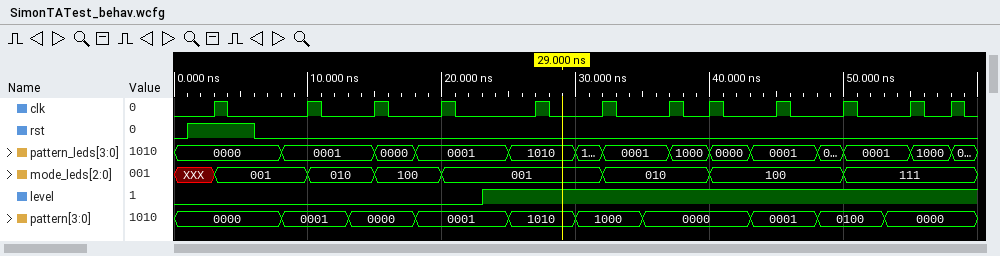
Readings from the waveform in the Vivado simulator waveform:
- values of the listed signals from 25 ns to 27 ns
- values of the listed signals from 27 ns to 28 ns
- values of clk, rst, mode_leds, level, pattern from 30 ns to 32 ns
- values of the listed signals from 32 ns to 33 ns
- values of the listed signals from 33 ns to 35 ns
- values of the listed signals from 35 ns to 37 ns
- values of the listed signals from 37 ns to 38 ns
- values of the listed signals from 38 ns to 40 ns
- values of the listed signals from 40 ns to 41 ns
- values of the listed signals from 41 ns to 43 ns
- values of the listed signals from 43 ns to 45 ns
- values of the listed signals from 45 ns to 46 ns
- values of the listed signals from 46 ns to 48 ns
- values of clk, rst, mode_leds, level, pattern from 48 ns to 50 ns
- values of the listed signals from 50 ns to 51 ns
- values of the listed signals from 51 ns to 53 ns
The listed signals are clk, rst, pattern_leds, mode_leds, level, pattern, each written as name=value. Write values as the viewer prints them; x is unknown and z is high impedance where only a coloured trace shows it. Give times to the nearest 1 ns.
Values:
clk=0, rst=0, pattern_leds=1010, mode_leds=001, level=1, pattern=1010
clk=1, rst=0, pattern_leds=1010, mode_leds=001, level=1, pattern=1010
clk=0, rst=0, mode_leds=001, level=1, pattern=1000
clk=1, rst=0, pattern_leds=0001, mode_leds=010, level=1, pattern=1000
clk=0, rst=0, pattern_leds=0001, mode_leds=010, level=1, pattern=1000
clk=0, rst=0, pattern_leds=0001, mode_leds=010, level=1, pattern=0000
clk=1, rst=0, pattern_leds=1000, mode_leds=010, level=1, pattern=0000
clk=0, rst=0, pattern_leds=1000, mode_leds=010, level=1, pattern=0000
clk=1, rst=0, pattern_leds=0000, mode_leds=100, level=1, pattern=0000
clk=0, rst=0, pattern_leds=0000, mode_leds=100, level=1, pattern=0000
clk=0, rst=0, pattern_leds=0001, mode_leds=100, level=1, pattern=0001
clk=1, rst=0, pattern_leds=0001, mode_leds=100, level=1, pattern=0001
clk=0, rst=0, pattern_leds=0001, mode_leds=100, level=1, pattern=0001
clk=0, rst=0, mode_leds=100, level=1, pattern=0100
clk=1, rst=0, pattern_leds=0001, mode_leds=111, level=1, pattern=0100
clk=0, rst=0, pattern_leds=0001, mode_leds=111, level=1, pattern=0100
